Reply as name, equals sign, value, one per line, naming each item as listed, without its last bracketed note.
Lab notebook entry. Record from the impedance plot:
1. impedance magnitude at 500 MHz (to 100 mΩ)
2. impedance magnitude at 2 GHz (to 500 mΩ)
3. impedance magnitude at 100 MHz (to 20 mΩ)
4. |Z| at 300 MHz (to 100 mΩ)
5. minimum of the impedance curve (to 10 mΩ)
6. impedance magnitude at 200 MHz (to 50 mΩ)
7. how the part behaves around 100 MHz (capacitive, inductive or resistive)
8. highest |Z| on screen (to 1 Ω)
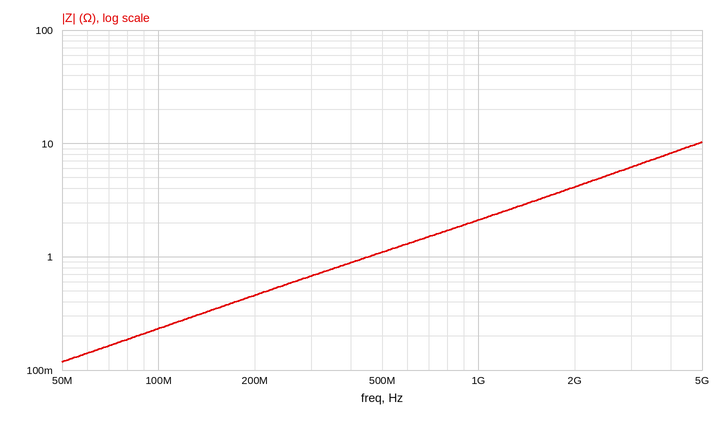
impedance magnitude at 500 MHz = 1.1 Ω
impedance magnitude at 2 GHz = 4.0 Ω
impedance magnitude at 100 MHz = 240 mΩ
|Z| at 300 MHz = 700 mΩ
minimum of the impedance curve = 120 mΩ
impedance magnitude at 200 MHz = 450 mΩ
how the part behaves around 100 MHz = inductive
highest |Z| on screen = 10 Ω
